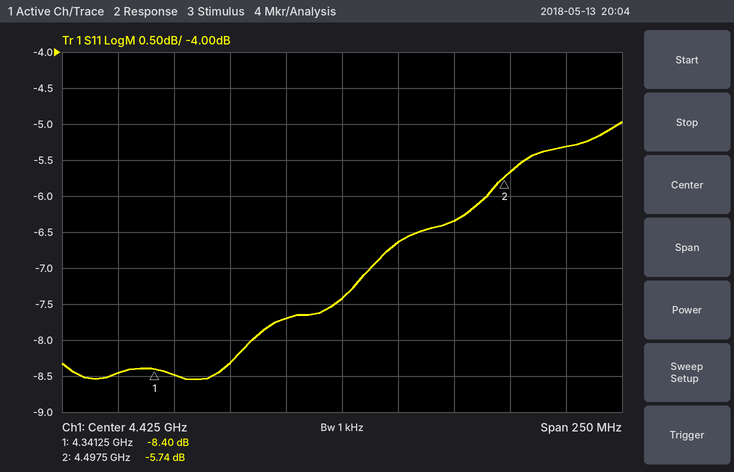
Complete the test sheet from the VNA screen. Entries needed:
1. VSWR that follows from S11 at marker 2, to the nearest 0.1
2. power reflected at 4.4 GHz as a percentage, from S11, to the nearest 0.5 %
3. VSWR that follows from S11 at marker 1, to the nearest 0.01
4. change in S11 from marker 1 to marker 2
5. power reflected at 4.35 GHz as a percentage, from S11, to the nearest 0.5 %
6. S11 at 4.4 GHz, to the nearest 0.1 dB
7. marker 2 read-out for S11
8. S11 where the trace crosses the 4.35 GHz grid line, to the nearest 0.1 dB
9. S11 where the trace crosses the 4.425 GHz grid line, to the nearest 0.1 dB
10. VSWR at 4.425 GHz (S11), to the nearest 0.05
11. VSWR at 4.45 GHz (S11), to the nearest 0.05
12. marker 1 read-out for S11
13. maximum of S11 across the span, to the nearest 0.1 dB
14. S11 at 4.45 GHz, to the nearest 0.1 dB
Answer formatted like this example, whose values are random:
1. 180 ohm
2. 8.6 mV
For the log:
1. 3.1
2. 17.0 %
3. 2.23
4. 2.66 dB
5. 14.0 %
6. -7.7 dB
7. -5.74 dB
8. -8.5 dB
9. -7.4 dB
10. 2.50
11. 2.75
12. -8.40 dB
13. -5.0 dB
14. -6.6 dB
